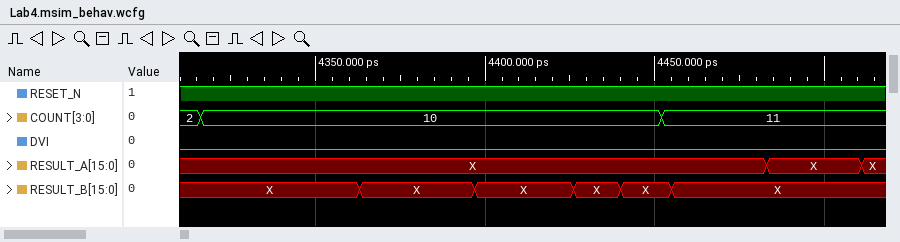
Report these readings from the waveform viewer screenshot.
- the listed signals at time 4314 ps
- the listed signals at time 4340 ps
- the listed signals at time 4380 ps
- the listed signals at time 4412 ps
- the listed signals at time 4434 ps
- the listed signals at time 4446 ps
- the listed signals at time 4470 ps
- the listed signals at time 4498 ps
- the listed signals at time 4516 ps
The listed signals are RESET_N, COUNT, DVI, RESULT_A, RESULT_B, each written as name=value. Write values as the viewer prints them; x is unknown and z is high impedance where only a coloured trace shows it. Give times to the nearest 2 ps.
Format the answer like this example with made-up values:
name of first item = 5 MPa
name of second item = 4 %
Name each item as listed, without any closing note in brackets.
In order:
the listed signals at time 4314 ps = RESET_N=1, COUNT=2, DVI=0, RESULT_A=X, RESULT_B=X
the listed signals at time 4340 ps = RESET_N=1, COUNT=10, DVI=0, RESULT_A=X, RESULT_B=X
the listed signals at time 4380 ps = RESET_N=1, COUNT=10, DVI=0, RESULT_A=X, RESULT_B=X
the listed signals at time 4412 ps = RESET_N=1, COUNT=10, DVI=0, RESULT_A=X, RESULT_B=X
the listed signals at time 4434 ps = RESET_N=1, COUNT=10, DVI=0, RESULT_A=X, RESULT_B=X
the listed signals at time 4446 ps = RESET_N=1, COUNT=10, DVI=0, RESULT_A=X, RESULT_B=X
the listed signals at time 4470 ps = RESET_N=1, COUNT=11, DVI=0, RESULT_A=X, RESULT_B=X
the listed signals at time 4498 ps = RESET_N=1, COUNT=11, DVI=0, RESULT_A=X, RESULT_B=X
the listed signals at time 4516 ps = RESET_N=1, COUNT=11, DVI=0, RESULT_A=X, RESULT_B=X
